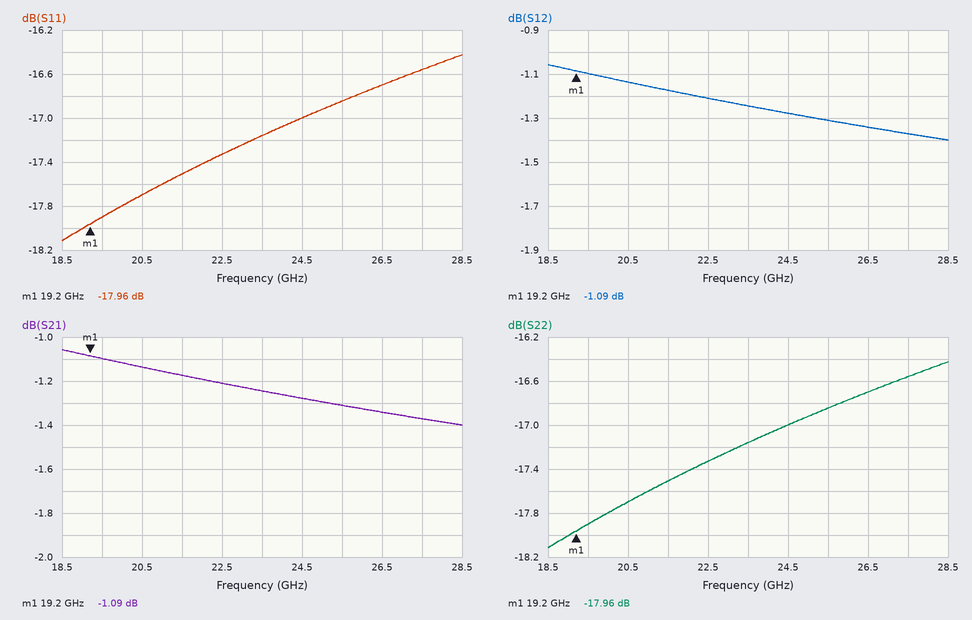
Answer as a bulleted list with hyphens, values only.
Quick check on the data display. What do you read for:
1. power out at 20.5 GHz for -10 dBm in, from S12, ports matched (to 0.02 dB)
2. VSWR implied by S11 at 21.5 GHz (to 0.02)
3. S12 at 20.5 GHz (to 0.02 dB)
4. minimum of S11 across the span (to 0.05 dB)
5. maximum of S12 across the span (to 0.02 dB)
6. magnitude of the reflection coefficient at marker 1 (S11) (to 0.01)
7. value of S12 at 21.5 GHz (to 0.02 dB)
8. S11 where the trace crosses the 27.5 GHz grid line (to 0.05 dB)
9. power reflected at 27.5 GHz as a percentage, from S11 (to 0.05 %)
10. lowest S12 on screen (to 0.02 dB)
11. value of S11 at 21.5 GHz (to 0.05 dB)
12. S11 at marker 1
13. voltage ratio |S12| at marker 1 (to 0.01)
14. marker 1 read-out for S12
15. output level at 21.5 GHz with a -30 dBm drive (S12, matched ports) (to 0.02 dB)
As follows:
- -11.14 dBm
- 1.30
- -1.14 dB
- -18.10 dB
- -1.06 dB
- 0.13
- -1.18 dB
- -16.55 dB
- 2.20 %
- -1.40 dB
- -17.50 dB
- -17.96 dB
- 0.88
- -1.09 dB
- -31.18 dBm
